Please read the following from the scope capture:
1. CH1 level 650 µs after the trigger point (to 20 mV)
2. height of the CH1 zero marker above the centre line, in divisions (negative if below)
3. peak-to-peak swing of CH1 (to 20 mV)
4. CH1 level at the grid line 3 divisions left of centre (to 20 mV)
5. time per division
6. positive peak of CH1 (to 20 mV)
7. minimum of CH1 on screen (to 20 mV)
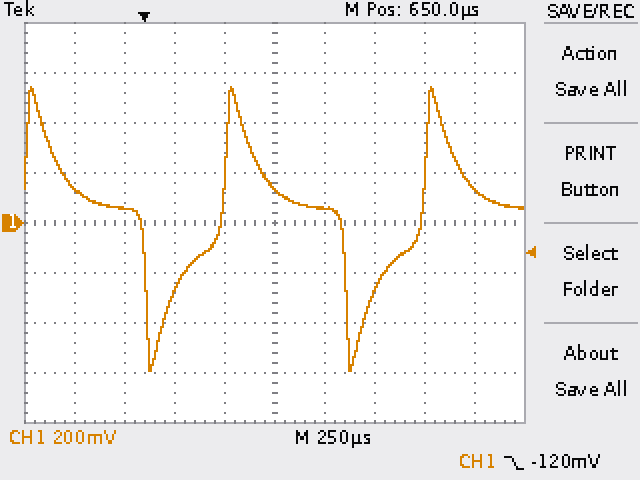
140 mV
0.0 div
1.14 V
60 mV
250 µs
540 mV
-600 mV
